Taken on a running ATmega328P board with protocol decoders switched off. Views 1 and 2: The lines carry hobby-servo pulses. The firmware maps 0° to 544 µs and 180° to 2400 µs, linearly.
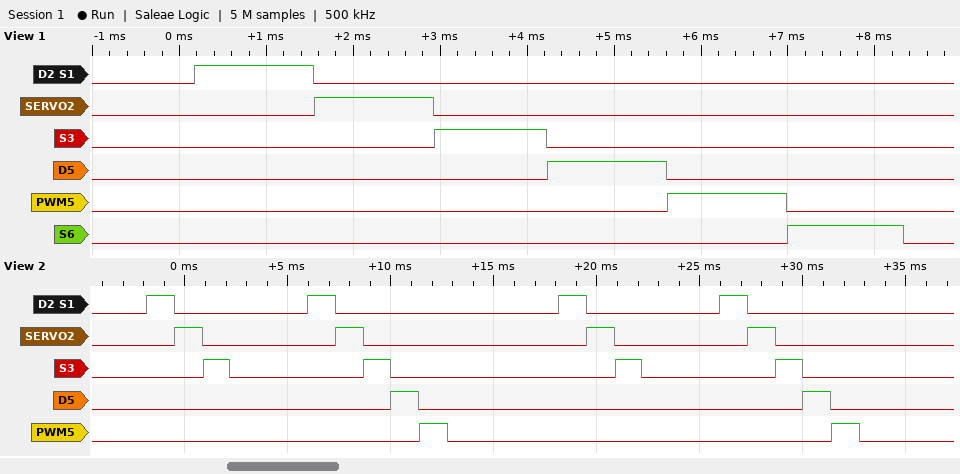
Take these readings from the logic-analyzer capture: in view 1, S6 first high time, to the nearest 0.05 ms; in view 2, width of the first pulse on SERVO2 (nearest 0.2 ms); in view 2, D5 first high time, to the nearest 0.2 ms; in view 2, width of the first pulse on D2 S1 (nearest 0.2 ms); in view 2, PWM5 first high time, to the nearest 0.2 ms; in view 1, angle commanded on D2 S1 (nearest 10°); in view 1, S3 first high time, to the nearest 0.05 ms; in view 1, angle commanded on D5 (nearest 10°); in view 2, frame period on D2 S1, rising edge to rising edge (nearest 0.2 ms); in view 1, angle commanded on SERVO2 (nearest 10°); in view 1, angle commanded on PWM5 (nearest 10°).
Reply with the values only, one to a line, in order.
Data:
1.35 ms
1.4 ms
1.4 ms
1.4 ms
1.4 ms
80°
1.30 ms
80°
7.8 ms
80°
80°
